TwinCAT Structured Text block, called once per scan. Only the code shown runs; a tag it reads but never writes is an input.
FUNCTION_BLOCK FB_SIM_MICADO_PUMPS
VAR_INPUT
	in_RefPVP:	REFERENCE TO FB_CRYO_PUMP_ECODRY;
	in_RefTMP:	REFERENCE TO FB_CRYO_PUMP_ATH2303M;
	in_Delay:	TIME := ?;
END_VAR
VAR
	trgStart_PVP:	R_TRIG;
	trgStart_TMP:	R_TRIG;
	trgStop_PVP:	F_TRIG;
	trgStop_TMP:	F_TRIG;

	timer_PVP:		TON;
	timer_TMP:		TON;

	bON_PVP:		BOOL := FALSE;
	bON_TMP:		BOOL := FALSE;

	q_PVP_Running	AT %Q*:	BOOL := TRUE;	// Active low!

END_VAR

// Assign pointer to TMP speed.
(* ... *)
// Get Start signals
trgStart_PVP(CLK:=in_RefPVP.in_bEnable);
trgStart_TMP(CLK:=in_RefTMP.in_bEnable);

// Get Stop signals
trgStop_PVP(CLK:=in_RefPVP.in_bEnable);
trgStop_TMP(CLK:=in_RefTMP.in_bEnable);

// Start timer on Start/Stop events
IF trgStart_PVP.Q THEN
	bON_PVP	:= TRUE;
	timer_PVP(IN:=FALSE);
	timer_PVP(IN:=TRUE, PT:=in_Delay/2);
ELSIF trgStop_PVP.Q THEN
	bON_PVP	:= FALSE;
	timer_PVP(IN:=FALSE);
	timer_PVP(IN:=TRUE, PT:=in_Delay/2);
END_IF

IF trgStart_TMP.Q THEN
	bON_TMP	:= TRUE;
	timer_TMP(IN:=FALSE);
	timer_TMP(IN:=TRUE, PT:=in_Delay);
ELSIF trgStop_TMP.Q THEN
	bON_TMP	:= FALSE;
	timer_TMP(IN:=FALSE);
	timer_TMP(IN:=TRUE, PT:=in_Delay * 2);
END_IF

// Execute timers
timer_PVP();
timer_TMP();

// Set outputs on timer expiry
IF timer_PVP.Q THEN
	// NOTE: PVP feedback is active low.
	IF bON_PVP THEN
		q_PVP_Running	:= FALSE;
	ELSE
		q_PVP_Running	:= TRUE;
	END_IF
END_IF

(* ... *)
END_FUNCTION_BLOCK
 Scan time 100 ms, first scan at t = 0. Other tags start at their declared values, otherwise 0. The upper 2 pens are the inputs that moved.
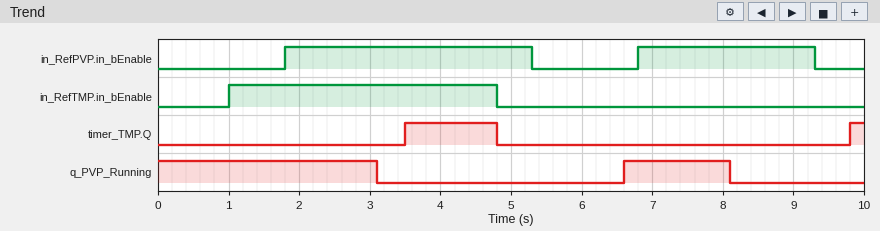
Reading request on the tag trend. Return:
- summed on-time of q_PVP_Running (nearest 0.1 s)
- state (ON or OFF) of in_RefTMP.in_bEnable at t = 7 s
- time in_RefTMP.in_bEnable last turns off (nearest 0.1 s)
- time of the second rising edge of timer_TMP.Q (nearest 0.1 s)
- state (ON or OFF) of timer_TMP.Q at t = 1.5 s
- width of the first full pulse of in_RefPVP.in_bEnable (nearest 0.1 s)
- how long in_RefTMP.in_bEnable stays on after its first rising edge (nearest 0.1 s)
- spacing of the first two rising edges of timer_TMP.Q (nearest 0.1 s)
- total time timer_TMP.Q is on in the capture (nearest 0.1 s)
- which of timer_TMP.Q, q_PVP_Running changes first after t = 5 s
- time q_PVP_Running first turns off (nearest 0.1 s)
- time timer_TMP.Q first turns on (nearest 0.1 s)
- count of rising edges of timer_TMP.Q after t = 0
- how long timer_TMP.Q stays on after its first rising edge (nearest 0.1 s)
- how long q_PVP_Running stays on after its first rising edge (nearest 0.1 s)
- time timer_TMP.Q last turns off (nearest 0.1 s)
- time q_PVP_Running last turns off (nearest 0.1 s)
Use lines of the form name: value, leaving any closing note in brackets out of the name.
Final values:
summed on-time of q_PVP_Running: 4.6 s
state (ON or OFF) of in_RefTMP.in_bEnable at t = 7 s: OFF
time in_RefTMP.in_bEnable last turns off: 4.8 s
time of the second rising edge of timer_TMP.Q: 9.8 s
state (ON or OFF) of timer_TMP.Q at t = 1.5 s: OFF
width of the first full pulse of in_RefPVP.in_bEnable: 3.5 s
how long in_RefTMP.in_bEnable stays on after its first rising edge: 3.8 s
spacing of the first two rising edges of timer_TMP.Q: 6.3 s
total time timer_TMP.Q is on in the capture: 1.5 s
which of timer_TMP.Q, q_PVP_Running changes first after t = 5 s: q_PVP_Running
time q_PVP_Running first turns off: 3.1 s
time timer_TMP.Q first turns on: 3.5 s
count of rising edges of timer_TMP.Q after t = 0: 2
how long timer_TMP.Q stays on after its first rising edge: 1.3 s
how long q_PVP_Running stays on after its first rising edge: 1.5 s
time timer_TMP.Q last turns off: 4.8 s
time q_PVP_Running last turns off: 8.1 s
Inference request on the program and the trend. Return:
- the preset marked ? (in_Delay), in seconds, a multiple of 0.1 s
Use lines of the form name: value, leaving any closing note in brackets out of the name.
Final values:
the preset marked ? (in_Delay), in seconds, a multiple of 0.1 s: 2.5 s
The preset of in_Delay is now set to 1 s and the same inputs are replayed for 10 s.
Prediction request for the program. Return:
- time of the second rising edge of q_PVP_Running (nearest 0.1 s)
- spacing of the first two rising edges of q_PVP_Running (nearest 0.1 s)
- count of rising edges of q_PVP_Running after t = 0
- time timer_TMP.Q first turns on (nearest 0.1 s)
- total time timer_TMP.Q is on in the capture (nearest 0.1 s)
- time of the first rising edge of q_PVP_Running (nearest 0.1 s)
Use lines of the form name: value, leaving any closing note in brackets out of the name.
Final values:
time of the second rising edge of q_PVP_Running: 9.8 s
spacing of the first two rising edges of q_PVP_Running: 4.0 s
count of rising edges of q_PVP_Running after t = 0: 2
time timer_TMP.Q first turns on: 2.0 s
total time timer_TMP.Q is on in the capture: 6.0 s
time of the first rising edge of q_PVP_Running: 5.8 s
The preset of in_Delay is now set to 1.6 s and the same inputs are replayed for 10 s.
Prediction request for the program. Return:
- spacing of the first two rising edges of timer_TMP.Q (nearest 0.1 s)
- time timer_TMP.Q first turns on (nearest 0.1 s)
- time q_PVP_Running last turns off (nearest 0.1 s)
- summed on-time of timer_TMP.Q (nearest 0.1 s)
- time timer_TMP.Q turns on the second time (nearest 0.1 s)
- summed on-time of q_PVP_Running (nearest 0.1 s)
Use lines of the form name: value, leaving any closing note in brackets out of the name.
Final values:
spacing of the first two rising edges of timer_TMP.Q: 5.4 s
time timer_TMP.Q first turns on: 2.6 s
time q_PVP_Running last turns off: 7.6 s
summed on-time of timer_TMP.Q: 4.2 s
time timer_TMP.Q turns on the second time: 8.0 s
summed on-time of q_PVP_Running: 4.1 s
